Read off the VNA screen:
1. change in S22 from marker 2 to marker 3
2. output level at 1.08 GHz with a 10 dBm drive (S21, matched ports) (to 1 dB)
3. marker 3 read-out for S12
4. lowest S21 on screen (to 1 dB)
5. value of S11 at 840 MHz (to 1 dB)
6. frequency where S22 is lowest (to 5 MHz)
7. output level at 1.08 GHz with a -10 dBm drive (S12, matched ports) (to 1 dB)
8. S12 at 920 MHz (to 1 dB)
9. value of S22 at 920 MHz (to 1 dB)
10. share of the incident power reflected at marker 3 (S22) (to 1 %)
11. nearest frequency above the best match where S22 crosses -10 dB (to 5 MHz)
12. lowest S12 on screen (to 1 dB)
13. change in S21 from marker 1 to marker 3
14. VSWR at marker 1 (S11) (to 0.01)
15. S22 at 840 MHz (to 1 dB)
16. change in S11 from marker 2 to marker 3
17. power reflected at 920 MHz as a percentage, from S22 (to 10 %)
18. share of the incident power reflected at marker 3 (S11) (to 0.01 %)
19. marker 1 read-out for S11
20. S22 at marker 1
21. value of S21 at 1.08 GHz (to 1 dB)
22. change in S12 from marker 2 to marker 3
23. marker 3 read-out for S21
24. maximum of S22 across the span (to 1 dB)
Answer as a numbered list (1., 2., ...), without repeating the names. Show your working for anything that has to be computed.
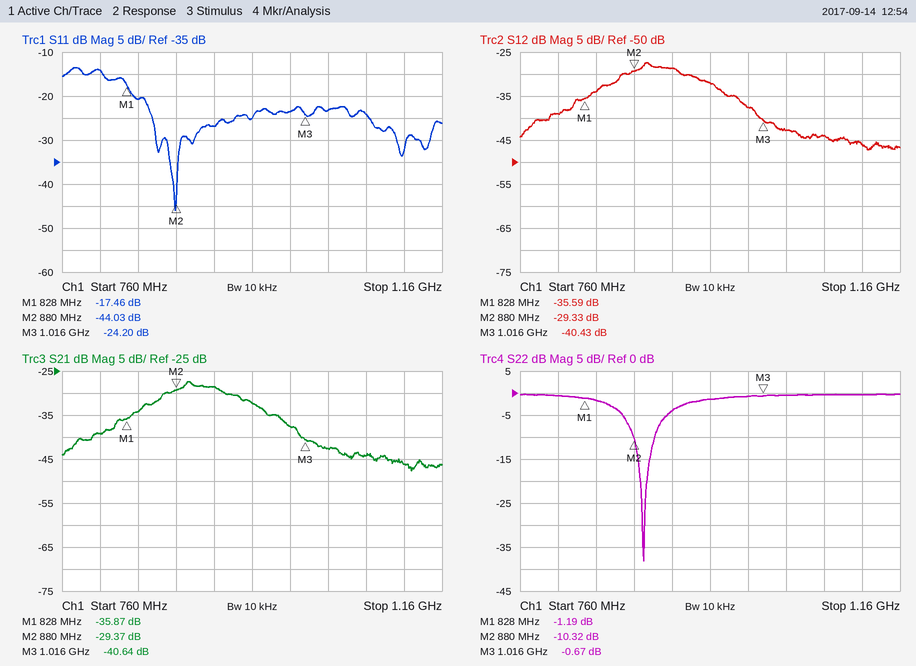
1. -0.67 − (-10.32) = 9.65 dB
2. 10 dBm + (-44 dB) = -34 dBm
3. -40.43 dB
4. -48 dB
5. -21 dB
6. 890 MHz
7. -10 dBm + (-44 dB) = -54 dBm
8. -29 dB
9. -4 dB
10. 10^(-0.67/10) ≈ 86 %
11. 900 MHz
12. -47 dB
13. -40.64 − (-35.87) = -4.77 dB
14. (1 + 0.1340)/(1 − 0.1340) ≈ 1.31
15. -2 dB
16. -24.2 − (-44.03) = 19.83 dB
17. 10^(-4/10) ≈ 40 %
18. 10^(-24.2/10) ≈ 0.38 %
19. -17.46 dB
20. -1.19 dB
21. -44 dB
22. -40.43 − (-29.33) = -11.10 dB
23. -40.64 dB
24. 0 dB
